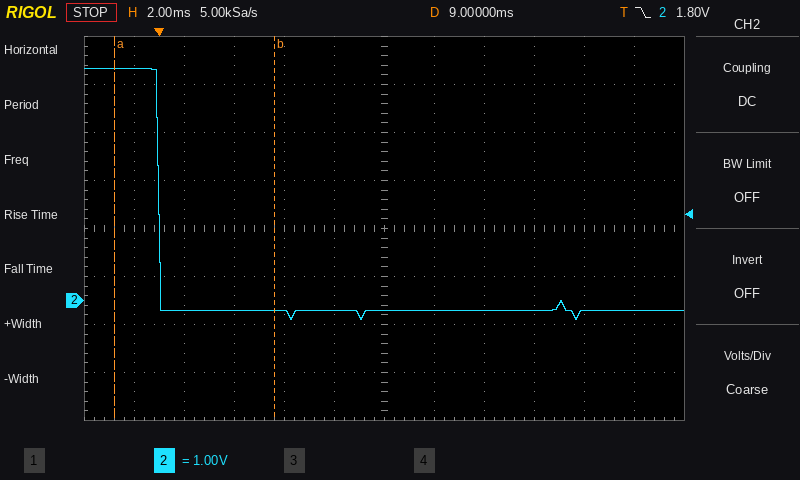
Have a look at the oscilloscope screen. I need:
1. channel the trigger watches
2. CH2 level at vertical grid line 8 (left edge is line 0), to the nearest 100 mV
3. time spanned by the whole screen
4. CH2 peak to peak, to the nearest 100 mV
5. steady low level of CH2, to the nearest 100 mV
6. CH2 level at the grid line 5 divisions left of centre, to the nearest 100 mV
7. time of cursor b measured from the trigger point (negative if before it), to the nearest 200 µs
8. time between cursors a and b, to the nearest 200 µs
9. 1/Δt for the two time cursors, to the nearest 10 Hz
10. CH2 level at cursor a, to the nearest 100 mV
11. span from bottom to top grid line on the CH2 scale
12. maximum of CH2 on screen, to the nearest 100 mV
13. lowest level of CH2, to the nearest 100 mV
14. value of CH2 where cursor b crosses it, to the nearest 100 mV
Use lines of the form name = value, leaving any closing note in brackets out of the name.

channel the trigger watches = CH2
CH2 level at vertical grid line 8 (left edge is line 0), to the nearest 100 mV = -200 mV
time spanned by the whole screen = 24 ms
CH2 peak to peak, to the nearest 100 mV = 5.2 V
steady low level of CH2, to the nearest 100 mV = -200 mV
CH2 level at the grid line 5 divisions left of centre, to the nearest 100 mV = 4.8 V
time of cursor b measured from the trigger point (negative if before it), to the nearest 200 µs = +4.6 ms
time between cursors a and b, to the nearest 200 µs = 6.4 ms
1/Δt for the two time cursors, to the nearest 10 Hz = 160 Hz
CH2 level at cursor a, to the nearest 100 mV = 4.8 V
span from bottom to top grid line on the CH2 scale = 8 V
maximum of CH2 on screen, to the nearest 100 mV = 4.8 V
lowest level of CH2, to the nearest 100 mV = -400 mV
value of CH2 where cursor b crosses it, to the nearest 100 mV = -200 mV
